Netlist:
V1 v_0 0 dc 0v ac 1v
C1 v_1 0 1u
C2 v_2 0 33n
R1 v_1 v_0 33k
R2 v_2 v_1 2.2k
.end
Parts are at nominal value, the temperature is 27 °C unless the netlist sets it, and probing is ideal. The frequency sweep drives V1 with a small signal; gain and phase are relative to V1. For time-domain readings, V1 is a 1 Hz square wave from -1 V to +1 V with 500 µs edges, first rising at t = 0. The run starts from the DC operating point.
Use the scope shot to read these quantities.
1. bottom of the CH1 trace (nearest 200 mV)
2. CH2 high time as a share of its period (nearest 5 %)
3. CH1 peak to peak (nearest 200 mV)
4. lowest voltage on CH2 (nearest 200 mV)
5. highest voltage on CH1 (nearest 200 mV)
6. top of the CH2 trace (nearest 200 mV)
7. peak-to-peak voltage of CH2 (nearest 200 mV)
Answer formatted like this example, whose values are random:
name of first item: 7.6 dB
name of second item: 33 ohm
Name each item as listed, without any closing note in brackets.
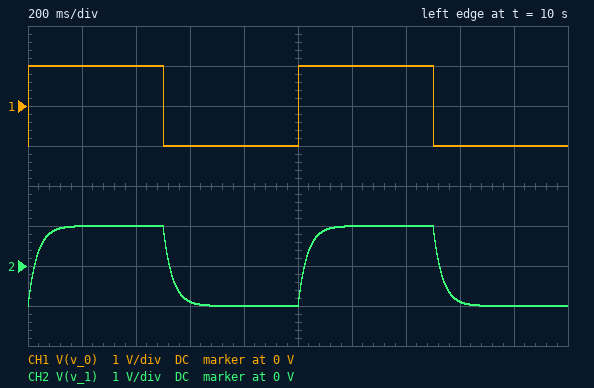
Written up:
bottom of the CH1 trace: -1.0 V
CH2 high time as a share of its period: 50 %
CH1 peak to peak: 2.0 V
lowest voltage on CH2: -1.0 V
highest voltage on CH1: 1.0 V
top of the CH2 trace: 1.0 V
peak-to-peak voltage of CH2: 2.0 V
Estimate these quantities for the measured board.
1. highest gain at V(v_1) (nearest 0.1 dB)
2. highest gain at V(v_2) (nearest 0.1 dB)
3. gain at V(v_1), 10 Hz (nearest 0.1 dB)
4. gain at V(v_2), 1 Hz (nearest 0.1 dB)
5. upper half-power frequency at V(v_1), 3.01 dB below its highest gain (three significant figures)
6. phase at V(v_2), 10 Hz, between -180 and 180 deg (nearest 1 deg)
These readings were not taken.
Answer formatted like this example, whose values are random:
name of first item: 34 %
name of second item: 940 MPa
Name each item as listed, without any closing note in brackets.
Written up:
highest gain at V(v_1): 0 dB
highest gain at V(v_2): 0 dB
gain at V(v_1), 10 Hz: -7.5 dB
gain at V(v_2), 1 Hz: -0.2 dB
upper half-power frequency at V(v_1), 3.01 dB below its highest gain: 4.67 Hz
phase at V(v_2), 10 Hz, between -180 and 180 deg: -65 deg
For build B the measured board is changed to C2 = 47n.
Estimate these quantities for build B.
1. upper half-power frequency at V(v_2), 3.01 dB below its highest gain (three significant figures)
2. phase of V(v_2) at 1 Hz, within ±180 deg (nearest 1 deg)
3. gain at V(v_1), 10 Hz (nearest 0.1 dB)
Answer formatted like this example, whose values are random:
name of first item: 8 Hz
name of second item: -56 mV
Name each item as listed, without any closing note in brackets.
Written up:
upper half-power frequency at V(v_2), 3.01 dB below its highest gain: 4.61 Hz
phase of V(v_2) at 1 Hz, within ±180 deg: -12 deg
gain at V(v_1), 10 Hz: -7.6 dB
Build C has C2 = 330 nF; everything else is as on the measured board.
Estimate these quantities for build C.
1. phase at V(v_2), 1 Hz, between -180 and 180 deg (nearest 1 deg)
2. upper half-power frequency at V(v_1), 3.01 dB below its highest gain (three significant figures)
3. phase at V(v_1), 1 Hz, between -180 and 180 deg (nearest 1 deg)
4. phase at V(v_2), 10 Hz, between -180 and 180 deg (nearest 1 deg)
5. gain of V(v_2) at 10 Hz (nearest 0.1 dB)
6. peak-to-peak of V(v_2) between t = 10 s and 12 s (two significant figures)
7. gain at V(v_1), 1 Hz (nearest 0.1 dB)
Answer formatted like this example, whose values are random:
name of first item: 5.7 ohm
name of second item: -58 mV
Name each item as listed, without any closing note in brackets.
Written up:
phase at V(v_2), 1 Hz, between -180 and 180 deg: -16 deg
upper half-power frequency at V(v_1), 3.01 dB below its highest gain: 3.61 Hz
phase at V(v_1), 1 Hz, between -180 and 180 deg: -15 deg
phase at V(v_2), 10 Hz, between -180 and 180 deg: -72 deg
gain of V(v_2) at 10 Hz: -9.4 dB
peak-to-peak of V(v_2) between t = 10 s and 12 s: 2.0 V
gain at V(v_1), 1 Hz: -0.3 dB
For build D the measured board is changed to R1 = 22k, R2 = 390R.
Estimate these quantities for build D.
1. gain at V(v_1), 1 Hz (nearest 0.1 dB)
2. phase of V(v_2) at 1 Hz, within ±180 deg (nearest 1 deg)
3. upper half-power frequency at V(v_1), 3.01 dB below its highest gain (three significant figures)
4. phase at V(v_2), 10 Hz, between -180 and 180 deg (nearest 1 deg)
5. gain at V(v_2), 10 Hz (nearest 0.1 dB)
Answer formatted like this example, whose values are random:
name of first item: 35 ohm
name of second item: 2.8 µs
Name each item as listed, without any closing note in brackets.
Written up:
gain at V(v_1), 1 Hz: -0.1 dB
phase of V(v_2) at 1 Hz, within ±180 deg: -8 deg
upper half-power frequency at V(v_1), 3.01 dB below its highest gain: 7.00 Hz
phase at V(v_2), 10 Hz, between -180 and 180 deg: -55 deg
gain at V(v_2), 10 Hz: -4.8 dB
